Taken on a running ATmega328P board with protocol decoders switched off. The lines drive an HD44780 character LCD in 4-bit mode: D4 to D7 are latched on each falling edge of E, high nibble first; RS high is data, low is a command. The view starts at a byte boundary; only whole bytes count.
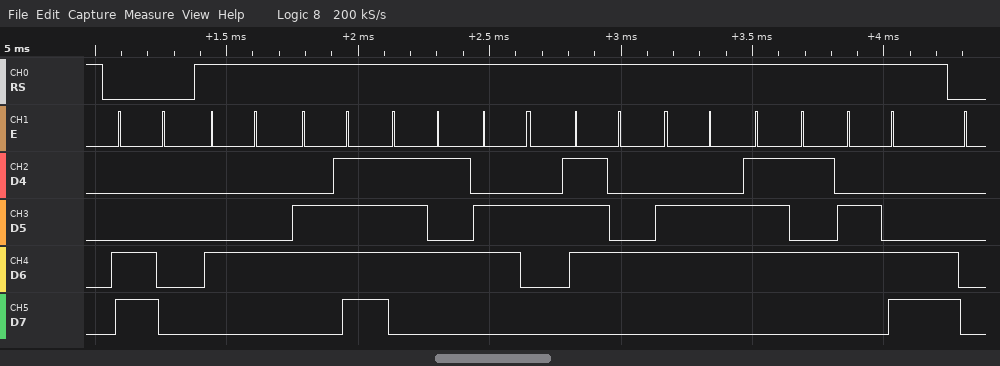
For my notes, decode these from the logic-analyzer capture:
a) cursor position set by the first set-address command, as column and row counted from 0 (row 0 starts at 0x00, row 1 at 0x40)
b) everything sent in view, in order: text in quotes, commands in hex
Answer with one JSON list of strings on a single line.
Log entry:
["column 0, row 1", "0xC0 \"Doubtful\""]
